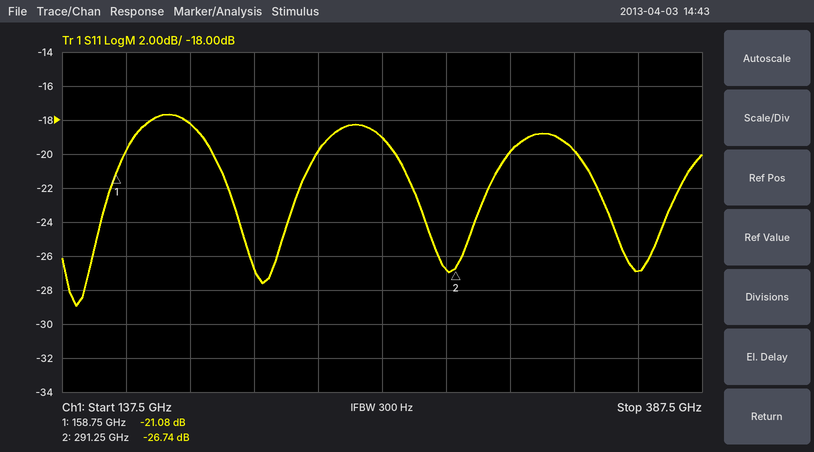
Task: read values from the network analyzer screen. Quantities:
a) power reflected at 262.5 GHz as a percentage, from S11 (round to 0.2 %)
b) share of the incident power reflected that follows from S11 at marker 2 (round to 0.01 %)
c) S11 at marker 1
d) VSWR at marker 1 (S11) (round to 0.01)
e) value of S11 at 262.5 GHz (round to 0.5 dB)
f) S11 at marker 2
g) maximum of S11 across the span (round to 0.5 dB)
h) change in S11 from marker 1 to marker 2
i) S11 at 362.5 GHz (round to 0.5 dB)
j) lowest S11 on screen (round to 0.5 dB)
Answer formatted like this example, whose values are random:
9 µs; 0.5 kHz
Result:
1.2 %; 0.21 %; -21.08 dB; 1.19; -19.0 dB; -26.74 dB; -17.5 dB; -5.66 dB; -27.0 dB; -29.0 dB
